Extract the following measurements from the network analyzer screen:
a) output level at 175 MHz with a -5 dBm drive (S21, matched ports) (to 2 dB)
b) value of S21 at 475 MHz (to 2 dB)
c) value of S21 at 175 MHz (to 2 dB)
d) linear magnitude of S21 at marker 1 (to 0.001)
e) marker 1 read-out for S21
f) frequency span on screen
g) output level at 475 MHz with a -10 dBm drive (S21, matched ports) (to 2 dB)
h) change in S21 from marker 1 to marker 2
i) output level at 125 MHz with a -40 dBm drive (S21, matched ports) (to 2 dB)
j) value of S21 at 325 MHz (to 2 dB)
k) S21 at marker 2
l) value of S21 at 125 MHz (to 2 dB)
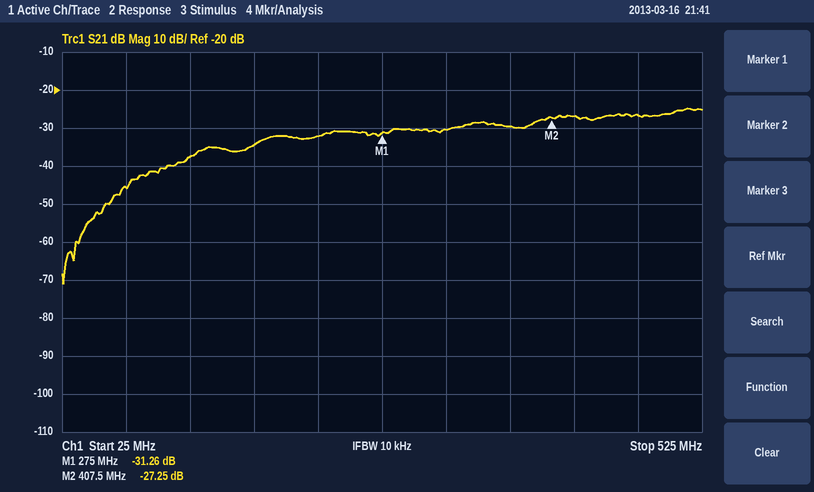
-40 dBm
-26 dB
-34 dB
0.027
-31.26 dB
500 MHz
-36 dBm
4.01 dB
-78 dBm
-30 dB
-27.25 dB
-38 dB
